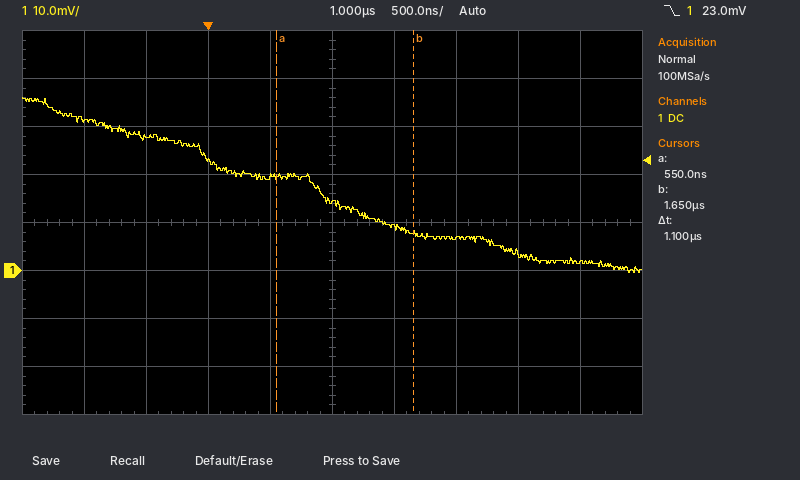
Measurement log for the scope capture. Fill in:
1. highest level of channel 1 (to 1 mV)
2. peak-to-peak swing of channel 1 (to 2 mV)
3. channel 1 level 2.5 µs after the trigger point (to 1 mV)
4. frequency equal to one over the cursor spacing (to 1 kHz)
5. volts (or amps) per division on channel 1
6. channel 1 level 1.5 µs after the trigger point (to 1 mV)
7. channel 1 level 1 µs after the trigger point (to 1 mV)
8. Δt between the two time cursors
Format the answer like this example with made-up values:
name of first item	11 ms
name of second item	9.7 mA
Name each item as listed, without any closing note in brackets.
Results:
highest level of channel 1	36 mV
peak-to-peak swing of channel 1	36 mV
channel 1 level 2.5 µs after the trigger point	4 mV
frequency equal to one over the cursor spacing	909 kHz
volts (or amps) per division on channel 1	10 mV
channel 1 level 1.5 µs after the trigger point	9 mV
channel 1 level 1 µs after the trigger point	14 mV
Δt between the two time cursors	1.1 µs
